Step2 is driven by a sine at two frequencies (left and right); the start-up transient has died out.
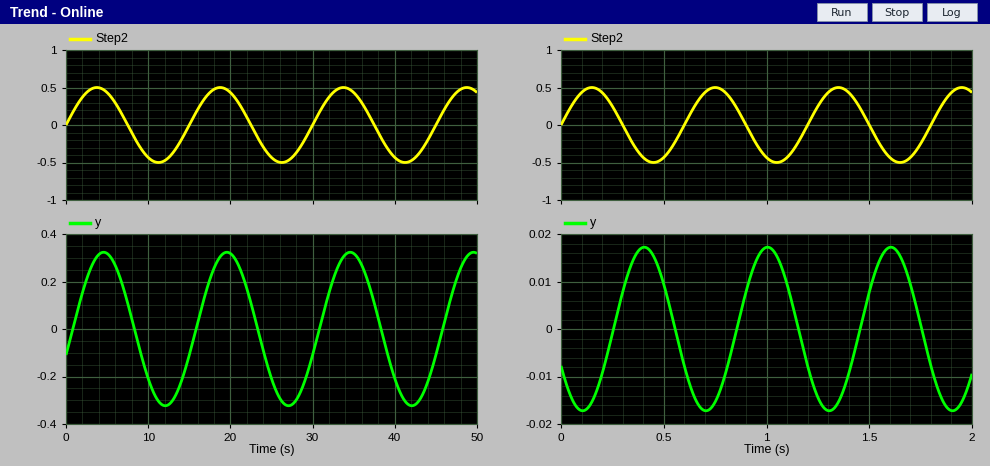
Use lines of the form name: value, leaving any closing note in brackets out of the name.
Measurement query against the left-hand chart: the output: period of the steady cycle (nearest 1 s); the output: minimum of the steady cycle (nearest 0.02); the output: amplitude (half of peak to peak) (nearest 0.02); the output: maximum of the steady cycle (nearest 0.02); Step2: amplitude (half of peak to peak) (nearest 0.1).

the output: period of the steady cycle: 15 s
the output: minimum of the steady cycle: -0.32
the output: amplitude (half of peak to peak): 0.32
the output: maximum of the steady cycle: 0.32
Step2: amplitude (half of peak to peak): 0.5
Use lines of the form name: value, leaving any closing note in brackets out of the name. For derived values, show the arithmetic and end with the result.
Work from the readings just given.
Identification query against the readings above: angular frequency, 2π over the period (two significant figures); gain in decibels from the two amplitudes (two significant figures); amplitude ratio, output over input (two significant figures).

angular frequency, 2π over the period: 2π / 15 = 0.42 rad/s
gain in decibels from the two amplitudes: 20 log10(0.32 / 0.5) = -3.9 dB
amplitude ratio, output over input: 0.32 / 0.5 = 0.64
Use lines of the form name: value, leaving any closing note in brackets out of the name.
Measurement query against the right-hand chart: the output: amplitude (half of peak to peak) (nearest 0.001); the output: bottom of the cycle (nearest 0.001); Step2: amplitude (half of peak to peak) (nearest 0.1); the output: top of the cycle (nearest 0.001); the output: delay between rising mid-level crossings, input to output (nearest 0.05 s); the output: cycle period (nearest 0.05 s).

the output: amplitude (half of peak to peak): 0.017
the output: bottom of the cycle: -0.017
Step2: amplitude (half of peak to peak): 0.5
the output: top of the cycle: 0.017
the output: delay between rising mid-level crossings, input to output: 0.25 s
the output: cycle period: 0.60 s
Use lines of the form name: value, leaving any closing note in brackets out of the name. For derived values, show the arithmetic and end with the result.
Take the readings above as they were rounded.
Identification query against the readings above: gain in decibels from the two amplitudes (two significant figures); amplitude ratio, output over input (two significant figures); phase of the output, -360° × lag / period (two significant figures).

gain in decibels from the two amplitudes: 20 log10(0.017 / 0.5) = -29 dB
amplitude ratio, output over input: 0.017 / 0.5 = 0.034
phase of the output, -360° × lag / period: -360 × 0.25 / 0.6 = -150°
